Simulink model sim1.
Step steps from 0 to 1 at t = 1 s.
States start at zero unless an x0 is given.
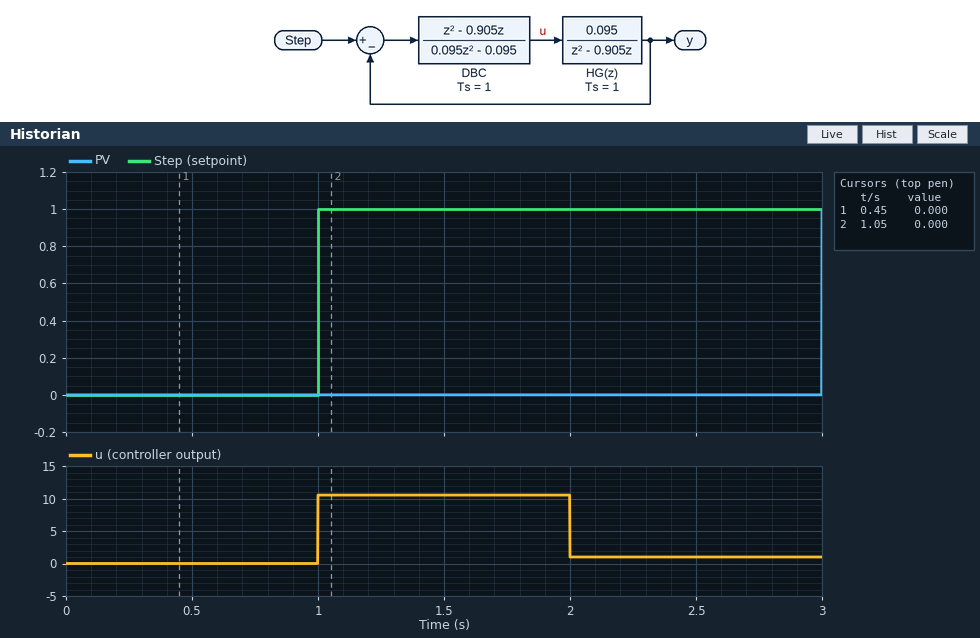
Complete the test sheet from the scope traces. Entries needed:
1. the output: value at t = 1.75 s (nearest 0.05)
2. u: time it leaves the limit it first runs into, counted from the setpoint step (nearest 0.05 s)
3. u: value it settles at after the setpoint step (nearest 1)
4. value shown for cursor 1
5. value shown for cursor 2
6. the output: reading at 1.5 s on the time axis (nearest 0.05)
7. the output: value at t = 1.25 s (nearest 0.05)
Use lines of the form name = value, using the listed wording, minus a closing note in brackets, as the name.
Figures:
the output: value at t = 1.75 s = 0.00
u: time it leaves the limit it first runs into, counted from the setpoint step = 1.00 s
u: value it settles at after the setpoint step = 1
value shown for cursor 1 = 0.000
value shown for cursor 2 = 0.000
the output: reading at 1.5 s on the time axis = 0.00
the output: value at t = 1.25 s = 0.00
